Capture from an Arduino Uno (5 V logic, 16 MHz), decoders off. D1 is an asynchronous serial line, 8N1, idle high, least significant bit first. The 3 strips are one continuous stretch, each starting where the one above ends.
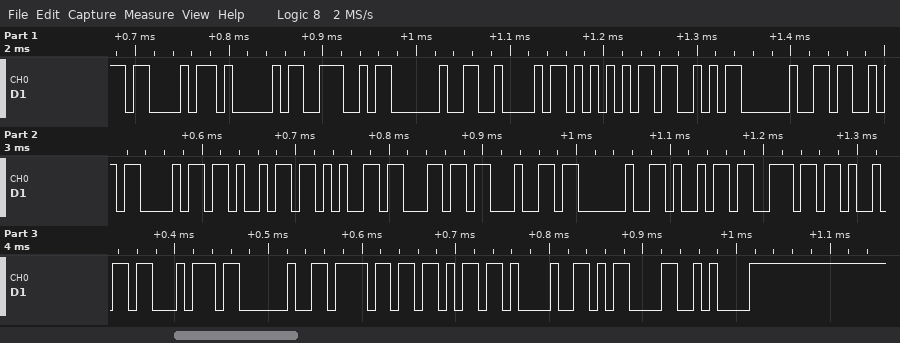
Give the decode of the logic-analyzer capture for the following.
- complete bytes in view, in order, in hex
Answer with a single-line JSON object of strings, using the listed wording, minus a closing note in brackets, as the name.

{"complete bytes in view, in order, in hex": "0x43 0x41 0x4E 0x20 0x42 0x55 0x53 0x20 0x53 0x68 0x69 0x65 0x6C 0x64 0x20 0x69 0x6E 0x69 0x74 0x20 0x6F 0x6B 0x21 0x0D 0x0A"}
